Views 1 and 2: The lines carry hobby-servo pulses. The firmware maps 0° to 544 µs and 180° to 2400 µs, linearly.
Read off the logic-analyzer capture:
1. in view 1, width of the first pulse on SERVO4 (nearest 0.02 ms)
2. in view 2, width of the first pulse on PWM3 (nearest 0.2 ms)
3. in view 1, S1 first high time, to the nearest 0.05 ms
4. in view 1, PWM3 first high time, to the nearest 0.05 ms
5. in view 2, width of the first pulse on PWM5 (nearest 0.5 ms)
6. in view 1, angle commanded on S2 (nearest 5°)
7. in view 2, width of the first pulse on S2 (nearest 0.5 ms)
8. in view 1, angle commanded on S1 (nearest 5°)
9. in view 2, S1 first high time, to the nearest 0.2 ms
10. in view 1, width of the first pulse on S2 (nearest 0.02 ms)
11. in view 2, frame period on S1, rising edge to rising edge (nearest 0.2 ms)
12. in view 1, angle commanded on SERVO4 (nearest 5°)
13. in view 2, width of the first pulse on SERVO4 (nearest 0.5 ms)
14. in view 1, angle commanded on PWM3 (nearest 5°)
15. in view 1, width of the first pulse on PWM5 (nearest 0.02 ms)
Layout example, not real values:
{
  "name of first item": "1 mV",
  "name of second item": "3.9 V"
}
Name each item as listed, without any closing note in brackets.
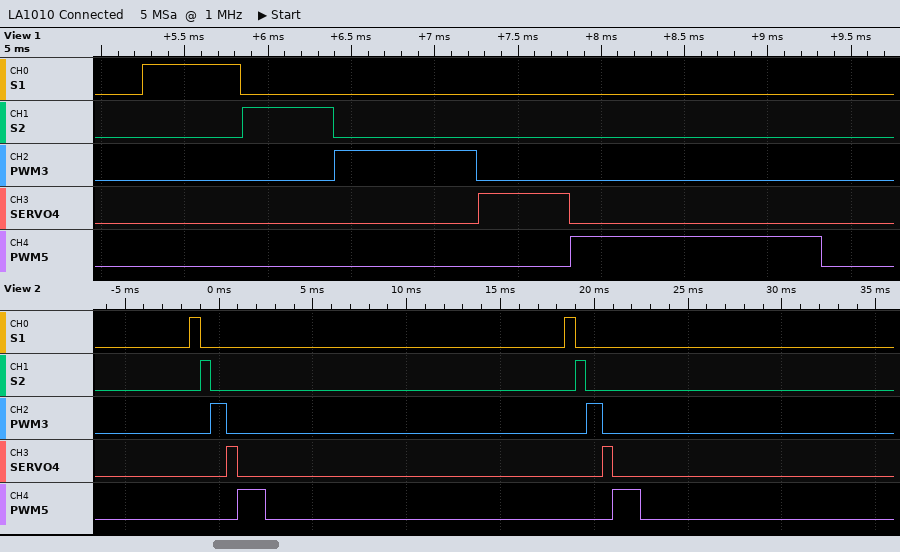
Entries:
{
  "in view 1, width of the first pulse on SERVO4": "0.54 ms",
  "in view 2, width of the first pulse on PWM3": "0.8 ms",
  "in view 1, S1 first high time, to the nearest 0.05 ms": "0.60 ms",
  "in view 1, PWM3 first high time, to the nearest 0.05 ms": "0.85 ms",
  "in view 2, width of the first pulse on PWM5": "1.5 ms",
  "in view 1, angle commanded on S2": "0°",
  "in view 2, width of the first pulse on S2": "0.5 ms",
  "in view 1, angle commanded on S1": "5°",
  "in view 2, S1 first high time, to the nearest 0.2 ms": "0.6 ms",
  "in view 1, width of the first pulse on S2": "0.54 ms",
  "in view 2, frame period on S1, rising edge to rising edge": "20.0 ms",
  "in view 1, angle commanded on SERVO4": "0°",
  "in view 2, width of the first pulse on SERVO4": "0.5 ms",
  "in view 1, angle commanded on PWM3": "30°",
  "in view 1, width of the first pulse on PWM5": "1.50 ms"
}
